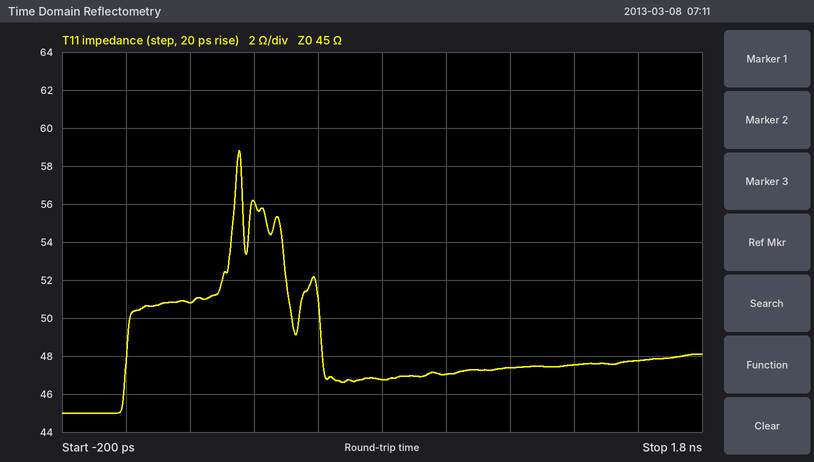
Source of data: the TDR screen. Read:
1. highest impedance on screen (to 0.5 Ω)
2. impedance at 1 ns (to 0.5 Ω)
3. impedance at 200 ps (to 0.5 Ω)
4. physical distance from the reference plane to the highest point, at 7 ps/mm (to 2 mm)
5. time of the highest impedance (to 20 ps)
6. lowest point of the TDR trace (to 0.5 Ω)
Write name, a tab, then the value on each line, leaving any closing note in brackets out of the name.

highest impedance on screen	59.0 Ω
impedance at 1 ns	47.0 Ω
impedance at 200 ps	51.0 Ω
physical distance from the reference plane to the highest point, at 7 ps/mm	26 mm
time of the highest impedance	360 ps
lowest point of the TDR trace	45.0 Ω
